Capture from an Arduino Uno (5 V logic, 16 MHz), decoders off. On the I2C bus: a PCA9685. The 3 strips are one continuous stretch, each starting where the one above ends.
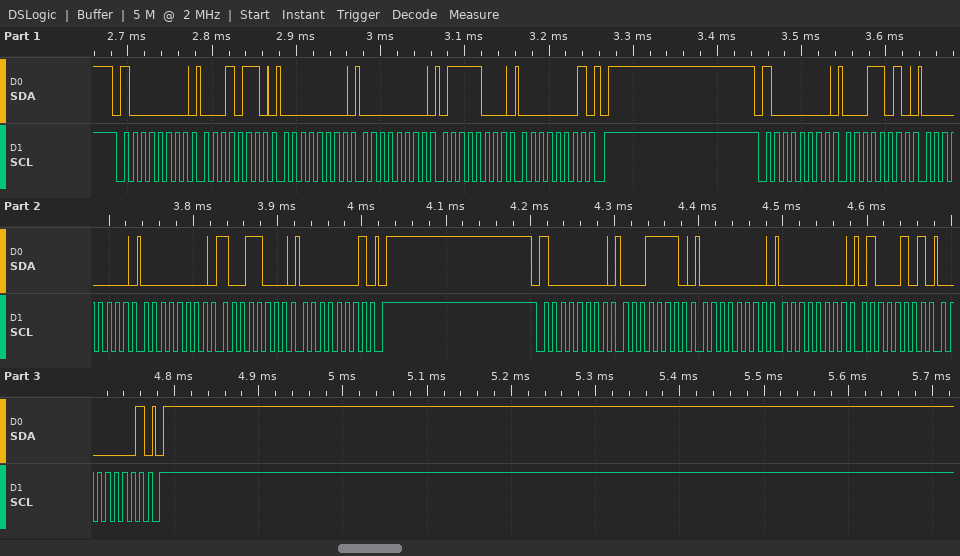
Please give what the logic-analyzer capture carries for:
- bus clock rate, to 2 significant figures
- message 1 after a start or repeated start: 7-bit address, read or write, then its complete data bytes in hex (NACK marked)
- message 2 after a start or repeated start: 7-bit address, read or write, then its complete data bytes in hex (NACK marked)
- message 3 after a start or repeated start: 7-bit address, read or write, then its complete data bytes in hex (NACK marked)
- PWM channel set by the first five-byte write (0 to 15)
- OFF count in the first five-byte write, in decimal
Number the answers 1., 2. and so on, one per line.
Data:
1. 100 kHz
2. 0x40 write: 16 00 00 78 01
3. 0x40 write: 1A 00 00 98 01
4. 0x40 write: 1E 00 00 45 01
5. 4
6. 376
